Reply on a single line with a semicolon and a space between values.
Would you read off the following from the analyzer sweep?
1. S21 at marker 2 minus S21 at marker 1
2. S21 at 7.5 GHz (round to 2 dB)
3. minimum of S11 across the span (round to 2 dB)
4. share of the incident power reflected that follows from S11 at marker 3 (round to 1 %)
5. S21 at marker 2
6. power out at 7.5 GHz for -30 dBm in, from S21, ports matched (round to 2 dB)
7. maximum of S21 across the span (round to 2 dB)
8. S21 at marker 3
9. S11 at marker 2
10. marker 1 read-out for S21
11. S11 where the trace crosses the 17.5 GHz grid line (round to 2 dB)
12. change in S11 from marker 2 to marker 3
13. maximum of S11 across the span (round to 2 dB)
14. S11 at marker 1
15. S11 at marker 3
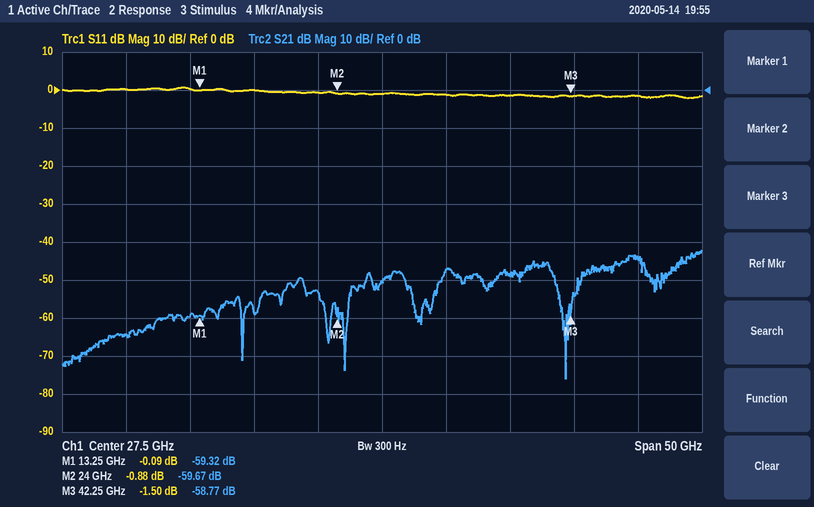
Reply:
-0.35 dB; -64 dB; -2 dB; 71 %; -59.67 dB; -94 dBm; -42 dB; -58.77 dB; -0.88 dB; -59.32 dB; 0 dB; -0.62 dB; 0 dB; -0.09 dB; -1.50 dB
